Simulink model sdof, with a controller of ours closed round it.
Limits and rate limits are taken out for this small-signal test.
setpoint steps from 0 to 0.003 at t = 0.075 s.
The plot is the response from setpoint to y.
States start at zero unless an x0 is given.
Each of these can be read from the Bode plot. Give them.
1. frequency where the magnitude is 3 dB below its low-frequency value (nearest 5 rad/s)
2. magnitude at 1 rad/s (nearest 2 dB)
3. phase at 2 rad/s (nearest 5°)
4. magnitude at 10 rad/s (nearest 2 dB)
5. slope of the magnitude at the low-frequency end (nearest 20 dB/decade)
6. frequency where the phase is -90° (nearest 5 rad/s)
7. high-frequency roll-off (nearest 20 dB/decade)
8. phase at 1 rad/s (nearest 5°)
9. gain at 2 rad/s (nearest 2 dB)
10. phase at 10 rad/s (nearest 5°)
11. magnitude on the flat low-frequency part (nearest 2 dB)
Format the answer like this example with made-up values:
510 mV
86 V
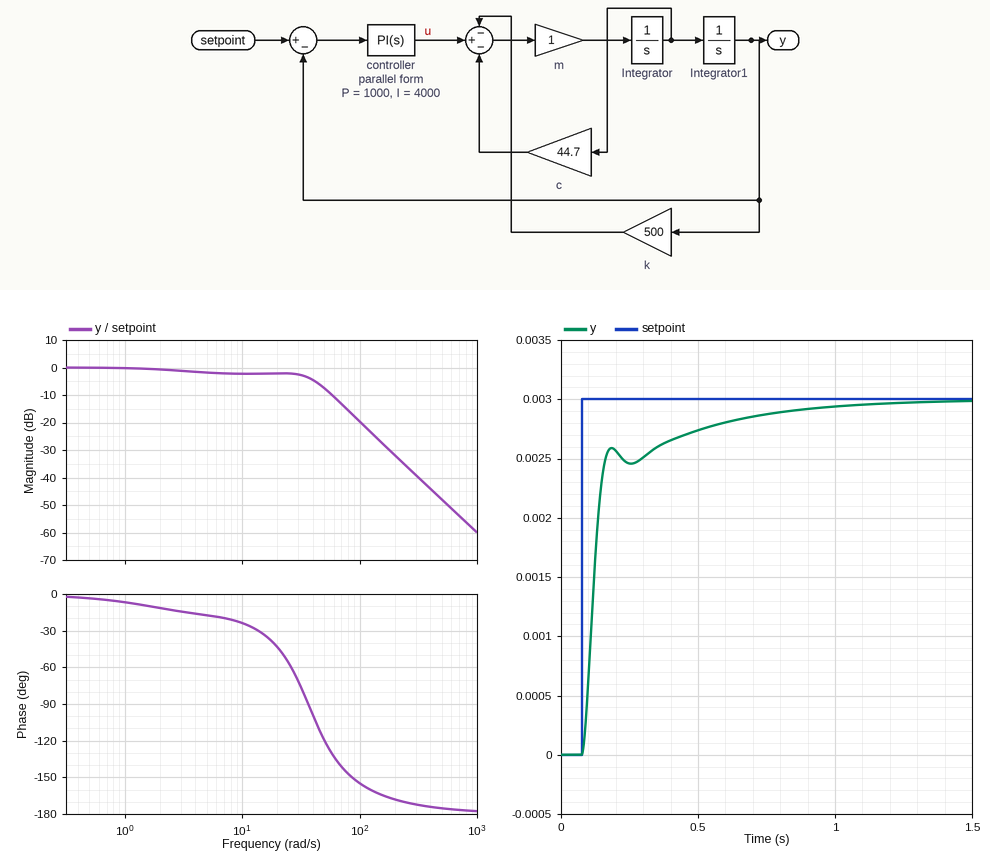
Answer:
35 rad/s
0 dB
-10°
-2 dB
0 dB/decade
35 rad/s
-40 dB/decade
-5°
0 dB
-25°
0 dB
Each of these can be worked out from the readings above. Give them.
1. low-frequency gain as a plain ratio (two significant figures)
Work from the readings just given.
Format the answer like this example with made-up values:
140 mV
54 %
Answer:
1.0
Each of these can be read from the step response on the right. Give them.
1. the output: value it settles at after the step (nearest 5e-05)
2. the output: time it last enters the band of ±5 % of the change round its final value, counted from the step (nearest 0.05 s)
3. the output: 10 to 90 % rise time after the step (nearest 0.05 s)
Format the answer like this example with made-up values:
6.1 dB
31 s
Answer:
0.00300
0.60 s
0.35 s
